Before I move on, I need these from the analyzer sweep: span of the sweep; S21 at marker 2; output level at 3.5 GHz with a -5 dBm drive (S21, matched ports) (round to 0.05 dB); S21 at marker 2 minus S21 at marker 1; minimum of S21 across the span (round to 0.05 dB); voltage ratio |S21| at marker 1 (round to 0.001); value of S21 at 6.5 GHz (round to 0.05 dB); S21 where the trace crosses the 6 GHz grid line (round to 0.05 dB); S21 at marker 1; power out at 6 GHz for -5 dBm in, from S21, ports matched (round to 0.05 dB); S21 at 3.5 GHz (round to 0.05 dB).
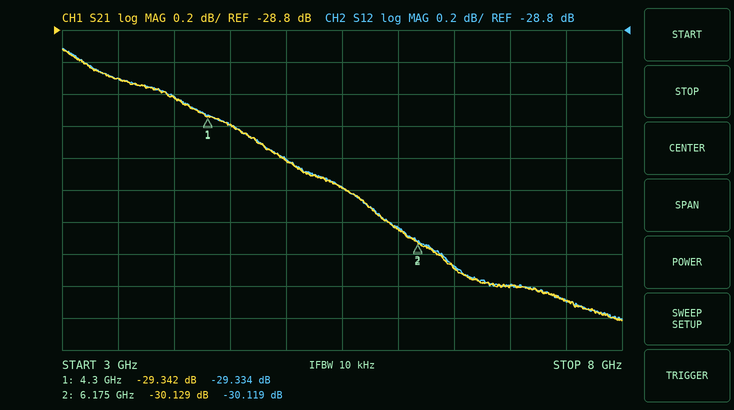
5 GHz
-30.129 dB
-34.10 dBm
-0.787 dB
-30.60 dB
0.034
-30.30 dB
-30.05 dB
-29.342 dB
-35.05 dBm
-29.10 dB
